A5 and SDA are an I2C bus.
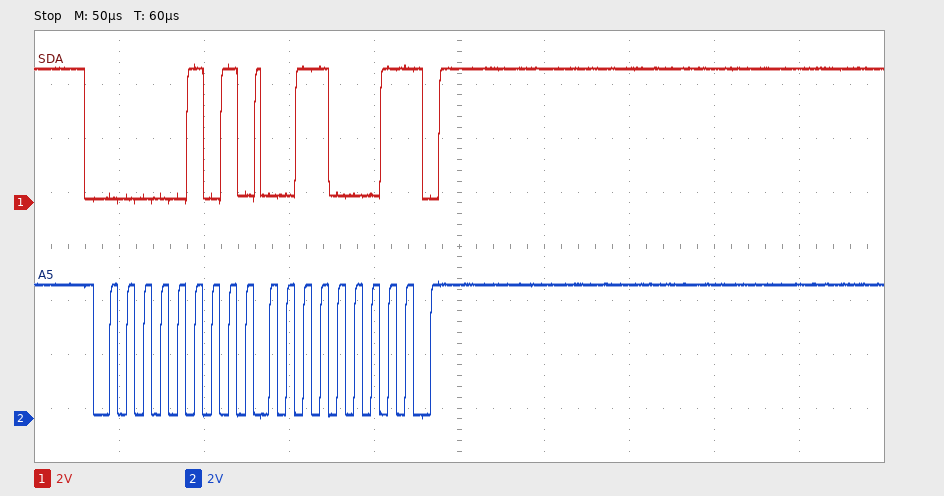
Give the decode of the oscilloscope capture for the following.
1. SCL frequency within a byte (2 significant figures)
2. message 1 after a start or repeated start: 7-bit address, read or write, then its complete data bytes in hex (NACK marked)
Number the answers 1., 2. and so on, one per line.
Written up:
1. 100 kHz
2. 0x02 read: 31 NACK
